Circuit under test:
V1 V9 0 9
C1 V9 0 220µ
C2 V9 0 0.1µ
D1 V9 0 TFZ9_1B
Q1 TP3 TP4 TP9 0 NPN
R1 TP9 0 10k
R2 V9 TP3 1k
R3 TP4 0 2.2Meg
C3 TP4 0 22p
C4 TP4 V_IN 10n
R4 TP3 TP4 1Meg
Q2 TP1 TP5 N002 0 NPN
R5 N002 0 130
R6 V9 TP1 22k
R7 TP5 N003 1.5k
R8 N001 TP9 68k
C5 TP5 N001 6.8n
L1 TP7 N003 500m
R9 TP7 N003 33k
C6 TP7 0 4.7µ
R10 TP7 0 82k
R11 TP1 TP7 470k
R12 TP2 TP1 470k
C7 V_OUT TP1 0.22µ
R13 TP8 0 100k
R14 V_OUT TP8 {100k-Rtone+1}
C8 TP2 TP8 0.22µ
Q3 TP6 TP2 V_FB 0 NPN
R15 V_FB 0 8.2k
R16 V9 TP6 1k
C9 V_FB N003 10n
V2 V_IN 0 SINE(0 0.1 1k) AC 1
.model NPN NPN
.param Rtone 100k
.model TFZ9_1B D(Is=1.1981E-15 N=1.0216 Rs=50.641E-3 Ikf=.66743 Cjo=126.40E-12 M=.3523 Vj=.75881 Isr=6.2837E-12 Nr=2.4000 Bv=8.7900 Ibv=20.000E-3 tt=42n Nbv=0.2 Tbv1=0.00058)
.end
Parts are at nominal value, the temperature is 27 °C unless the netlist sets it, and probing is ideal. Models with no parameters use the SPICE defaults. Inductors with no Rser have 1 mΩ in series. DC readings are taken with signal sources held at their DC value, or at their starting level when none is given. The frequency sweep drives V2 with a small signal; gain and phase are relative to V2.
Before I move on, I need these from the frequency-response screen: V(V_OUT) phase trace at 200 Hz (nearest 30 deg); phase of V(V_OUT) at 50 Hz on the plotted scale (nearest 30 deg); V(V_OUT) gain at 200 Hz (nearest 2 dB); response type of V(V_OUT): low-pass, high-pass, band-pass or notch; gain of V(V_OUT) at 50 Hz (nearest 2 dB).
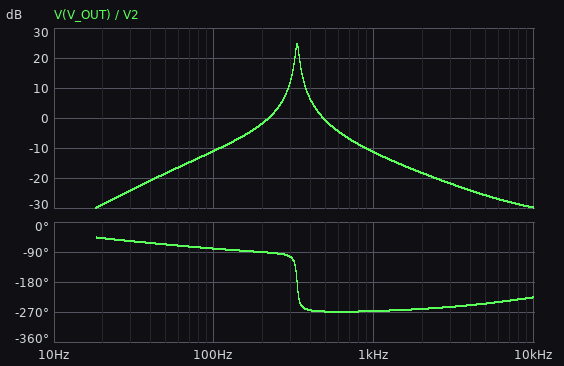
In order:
-90 deg
-60 deg
-2 dB
band-pass
-18 dB
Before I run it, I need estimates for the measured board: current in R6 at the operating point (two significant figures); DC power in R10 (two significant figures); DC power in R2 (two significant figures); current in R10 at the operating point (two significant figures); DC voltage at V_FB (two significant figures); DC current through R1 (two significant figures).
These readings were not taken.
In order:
150 µA
6.7 µW
98 µW
9.1 µA
3.1 V
310 µA
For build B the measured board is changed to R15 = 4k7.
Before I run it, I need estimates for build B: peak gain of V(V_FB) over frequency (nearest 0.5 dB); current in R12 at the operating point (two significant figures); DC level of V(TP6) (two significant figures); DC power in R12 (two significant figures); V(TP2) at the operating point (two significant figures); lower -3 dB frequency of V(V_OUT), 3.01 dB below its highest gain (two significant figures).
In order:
25.0 dB
5.2 µA
8.5 V
13 µW
3.2 V
330 Hz
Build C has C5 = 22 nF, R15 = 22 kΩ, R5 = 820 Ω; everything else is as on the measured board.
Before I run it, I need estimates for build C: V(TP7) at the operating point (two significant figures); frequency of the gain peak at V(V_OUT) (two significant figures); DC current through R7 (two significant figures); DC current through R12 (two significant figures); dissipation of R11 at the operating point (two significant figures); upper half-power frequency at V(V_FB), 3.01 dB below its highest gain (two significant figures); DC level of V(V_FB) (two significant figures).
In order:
820 mV
560 Hz
1.2 µA
2.0 µA
59 µW
580 Hz
4.4 V
